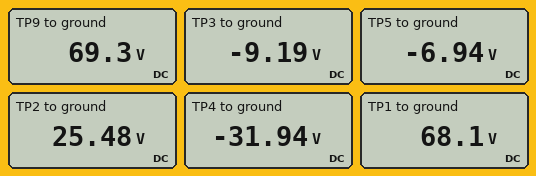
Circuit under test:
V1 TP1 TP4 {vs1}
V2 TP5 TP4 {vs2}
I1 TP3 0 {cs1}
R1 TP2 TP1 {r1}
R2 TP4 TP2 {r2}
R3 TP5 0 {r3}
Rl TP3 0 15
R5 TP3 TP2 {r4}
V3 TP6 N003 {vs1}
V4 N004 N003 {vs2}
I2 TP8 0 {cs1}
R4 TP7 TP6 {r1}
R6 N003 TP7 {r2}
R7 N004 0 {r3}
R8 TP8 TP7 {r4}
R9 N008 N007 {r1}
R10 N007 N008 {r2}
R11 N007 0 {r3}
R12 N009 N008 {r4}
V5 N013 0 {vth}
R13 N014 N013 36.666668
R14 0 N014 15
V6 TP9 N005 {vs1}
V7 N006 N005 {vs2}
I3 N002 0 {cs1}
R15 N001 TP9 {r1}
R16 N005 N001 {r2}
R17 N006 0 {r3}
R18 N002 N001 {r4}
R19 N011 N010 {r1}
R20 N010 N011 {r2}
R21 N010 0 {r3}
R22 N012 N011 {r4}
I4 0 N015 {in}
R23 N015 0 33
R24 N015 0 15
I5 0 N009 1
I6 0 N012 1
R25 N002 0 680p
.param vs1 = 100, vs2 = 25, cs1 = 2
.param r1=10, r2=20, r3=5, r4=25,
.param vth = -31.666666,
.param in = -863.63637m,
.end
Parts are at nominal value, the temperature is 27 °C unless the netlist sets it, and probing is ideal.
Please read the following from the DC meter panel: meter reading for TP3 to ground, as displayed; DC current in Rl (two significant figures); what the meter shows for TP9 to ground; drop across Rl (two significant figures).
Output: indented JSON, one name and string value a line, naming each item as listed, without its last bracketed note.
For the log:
{
  "meter reading for TP3 to ground, as displayed": "-9.19 V",
  "DC current in Rl": "610 mA",
  "what the meter shows for TP9 to ground": "69.3 V",
  "drop across Rl": "9.2 V"
}
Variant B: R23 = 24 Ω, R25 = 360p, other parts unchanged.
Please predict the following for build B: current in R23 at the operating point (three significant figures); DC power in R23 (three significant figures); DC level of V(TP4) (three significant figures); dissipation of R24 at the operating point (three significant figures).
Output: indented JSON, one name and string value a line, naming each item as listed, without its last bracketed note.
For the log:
{
  "current in R23 at the operating point": "332 mA",
  "DC power in R23": "2.65 W",
  "DC level of V(TP4)": "-31.9 V",
  "dissipation of R24 at the operating point": "4.24 W"
}
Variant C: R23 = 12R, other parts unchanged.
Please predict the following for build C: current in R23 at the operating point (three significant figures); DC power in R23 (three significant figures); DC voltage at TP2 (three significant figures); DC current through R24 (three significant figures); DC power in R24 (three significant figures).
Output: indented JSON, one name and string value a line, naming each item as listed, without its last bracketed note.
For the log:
{
  "current in R23 at the operating point": "480 mA",
  "DC power in R23": "2.76 W",
  "DC voltage at TP2": "25.5 V",
  "DC current through R24": "384 mA",
  "DC power in R24": "2.21 W"
}
